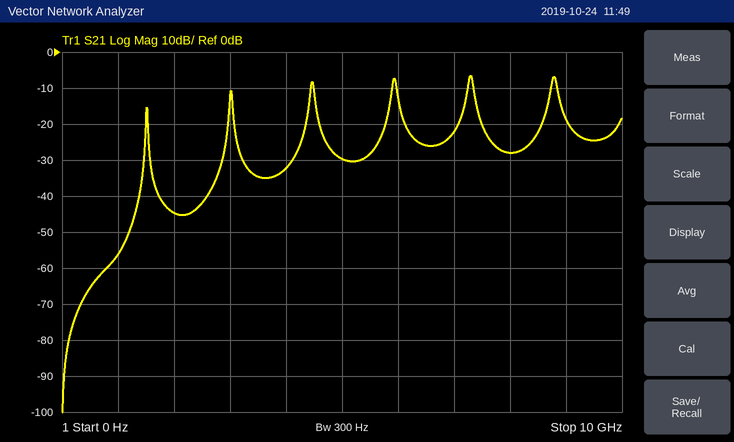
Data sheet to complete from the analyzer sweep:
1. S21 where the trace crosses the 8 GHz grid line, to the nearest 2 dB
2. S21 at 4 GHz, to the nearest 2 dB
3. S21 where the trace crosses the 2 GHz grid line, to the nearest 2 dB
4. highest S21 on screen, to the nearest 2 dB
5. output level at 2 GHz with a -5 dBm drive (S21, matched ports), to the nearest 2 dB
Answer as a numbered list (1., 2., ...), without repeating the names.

1. -28 dB
2. -32 dB
3. -44 dB
4. -6 dB
5. -50 dBm
